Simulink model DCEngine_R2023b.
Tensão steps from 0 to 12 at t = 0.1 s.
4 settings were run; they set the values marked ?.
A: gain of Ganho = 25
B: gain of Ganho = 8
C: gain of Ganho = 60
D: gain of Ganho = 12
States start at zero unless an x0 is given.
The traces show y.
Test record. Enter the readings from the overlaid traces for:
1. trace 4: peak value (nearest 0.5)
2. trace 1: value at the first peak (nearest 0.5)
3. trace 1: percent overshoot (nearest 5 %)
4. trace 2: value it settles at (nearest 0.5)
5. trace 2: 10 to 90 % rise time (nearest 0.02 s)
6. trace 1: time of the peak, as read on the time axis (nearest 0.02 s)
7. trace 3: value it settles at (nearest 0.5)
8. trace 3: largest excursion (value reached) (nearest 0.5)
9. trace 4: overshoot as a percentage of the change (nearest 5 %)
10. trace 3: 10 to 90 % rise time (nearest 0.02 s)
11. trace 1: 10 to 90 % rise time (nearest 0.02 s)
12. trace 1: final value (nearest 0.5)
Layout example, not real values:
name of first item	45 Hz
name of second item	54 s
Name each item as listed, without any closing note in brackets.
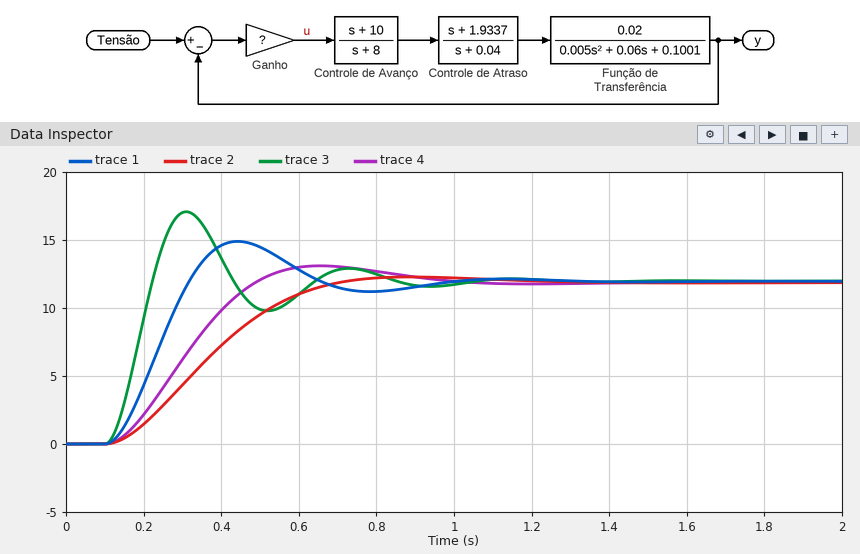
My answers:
trace 4: peak value	13.0
trace 1: value at the first peak	15.0
trace 1: percent overshoot	25 %
trace 2: value it settles at	12.0
trace 2: 10 to 90 % rise time	0.38 s
trace 1: time of the peak, as read on the time axis	0.44 s
trace 3: value it settles at	12.0
trace 3: largest excursion (value reached)	17.0
trace 4: overshoot as a percentage of the change	10 %
trace 3: 10 to 90 % rise time	0.08 s
trace 1: 10 to 90 % rise time	0.14 s
trace 1: final value	12.0
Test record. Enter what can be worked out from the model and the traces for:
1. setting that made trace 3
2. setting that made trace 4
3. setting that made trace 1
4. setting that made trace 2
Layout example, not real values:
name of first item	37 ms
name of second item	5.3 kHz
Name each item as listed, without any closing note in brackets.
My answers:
setting that made trace 3	C
setting that made trace 4	D
setting that made trace 1	A
setting that made trace 2	B
